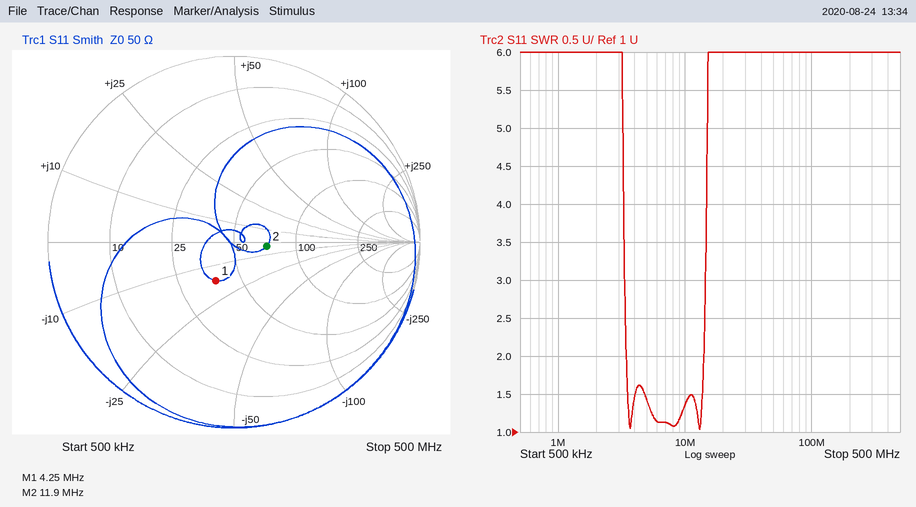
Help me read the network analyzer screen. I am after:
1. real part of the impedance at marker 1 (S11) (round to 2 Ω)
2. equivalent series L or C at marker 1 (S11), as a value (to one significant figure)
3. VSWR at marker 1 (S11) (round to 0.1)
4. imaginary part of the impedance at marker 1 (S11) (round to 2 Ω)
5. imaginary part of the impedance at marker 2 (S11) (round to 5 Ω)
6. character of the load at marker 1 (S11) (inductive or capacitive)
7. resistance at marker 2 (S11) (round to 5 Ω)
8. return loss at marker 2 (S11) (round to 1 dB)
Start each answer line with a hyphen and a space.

- 38 Ω
- 2 nF
- 1.6
- -16 Ω
- -5 Ω
- capacitive
- 70 Ω
- 15 dB
